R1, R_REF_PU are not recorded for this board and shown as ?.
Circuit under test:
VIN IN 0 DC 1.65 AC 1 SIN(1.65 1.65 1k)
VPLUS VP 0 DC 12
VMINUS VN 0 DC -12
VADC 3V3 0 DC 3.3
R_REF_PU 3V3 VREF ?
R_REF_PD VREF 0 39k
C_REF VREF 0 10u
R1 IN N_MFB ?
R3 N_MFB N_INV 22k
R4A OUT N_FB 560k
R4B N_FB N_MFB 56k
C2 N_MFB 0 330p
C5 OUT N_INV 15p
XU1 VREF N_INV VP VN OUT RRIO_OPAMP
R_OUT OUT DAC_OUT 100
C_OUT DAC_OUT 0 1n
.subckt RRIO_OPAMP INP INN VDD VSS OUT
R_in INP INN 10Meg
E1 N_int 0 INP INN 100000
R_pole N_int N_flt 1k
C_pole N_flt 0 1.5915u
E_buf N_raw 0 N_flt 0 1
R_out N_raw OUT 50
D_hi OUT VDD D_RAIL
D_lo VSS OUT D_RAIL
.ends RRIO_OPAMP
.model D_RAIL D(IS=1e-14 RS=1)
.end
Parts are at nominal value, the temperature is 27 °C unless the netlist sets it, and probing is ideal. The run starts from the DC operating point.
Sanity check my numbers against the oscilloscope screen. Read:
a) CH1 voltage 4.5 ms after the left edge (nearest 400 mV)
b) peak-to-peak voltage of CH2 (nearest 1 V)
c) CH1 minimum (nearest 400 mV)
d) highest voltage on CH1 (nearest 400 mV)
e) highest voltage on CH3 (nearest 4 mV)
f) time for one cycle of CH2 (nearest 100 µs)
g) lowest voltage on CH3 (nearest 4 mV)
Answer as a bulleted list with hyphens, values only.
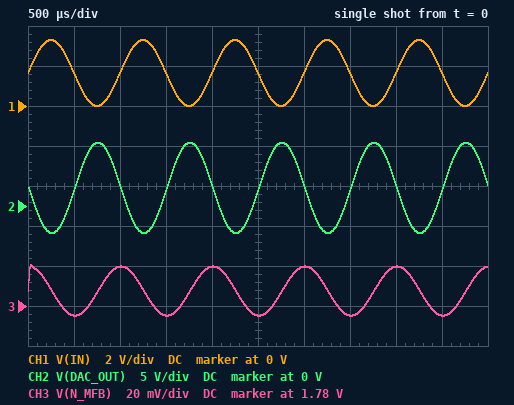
- 1.6 V
- 11 V
- 0 V
- 3.2 V
- 1.800 V
- 1.0 ms
- 1.776 V
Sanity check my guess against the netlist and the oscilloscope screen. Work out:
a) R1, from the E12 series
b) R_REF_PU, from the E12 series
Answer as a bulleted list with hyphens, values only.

- 180 kΩ
- 33 kΩ
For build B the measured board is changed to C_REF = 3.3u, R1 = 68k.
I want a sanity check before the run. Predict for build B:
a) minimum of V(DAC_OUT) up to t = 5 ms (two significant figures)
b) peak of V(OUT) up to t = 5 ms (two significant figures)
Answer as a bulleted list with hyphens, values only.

- -12 V
- 18 V
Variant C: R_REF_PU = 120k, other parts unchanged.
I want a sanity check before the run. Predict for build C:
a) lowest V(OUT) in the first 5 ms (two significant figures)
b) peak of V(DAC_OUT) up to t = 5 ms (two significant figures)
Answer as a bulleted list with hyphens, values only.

- -7.7 V
- 3.6 V
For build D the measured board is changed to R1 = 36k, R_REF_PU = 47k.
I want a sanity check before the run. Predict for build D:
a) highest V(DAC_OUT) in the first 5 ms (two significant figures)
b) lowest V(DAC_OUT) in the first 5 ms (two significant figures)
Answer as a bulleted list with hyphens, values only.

- 27 V
- -29 V
